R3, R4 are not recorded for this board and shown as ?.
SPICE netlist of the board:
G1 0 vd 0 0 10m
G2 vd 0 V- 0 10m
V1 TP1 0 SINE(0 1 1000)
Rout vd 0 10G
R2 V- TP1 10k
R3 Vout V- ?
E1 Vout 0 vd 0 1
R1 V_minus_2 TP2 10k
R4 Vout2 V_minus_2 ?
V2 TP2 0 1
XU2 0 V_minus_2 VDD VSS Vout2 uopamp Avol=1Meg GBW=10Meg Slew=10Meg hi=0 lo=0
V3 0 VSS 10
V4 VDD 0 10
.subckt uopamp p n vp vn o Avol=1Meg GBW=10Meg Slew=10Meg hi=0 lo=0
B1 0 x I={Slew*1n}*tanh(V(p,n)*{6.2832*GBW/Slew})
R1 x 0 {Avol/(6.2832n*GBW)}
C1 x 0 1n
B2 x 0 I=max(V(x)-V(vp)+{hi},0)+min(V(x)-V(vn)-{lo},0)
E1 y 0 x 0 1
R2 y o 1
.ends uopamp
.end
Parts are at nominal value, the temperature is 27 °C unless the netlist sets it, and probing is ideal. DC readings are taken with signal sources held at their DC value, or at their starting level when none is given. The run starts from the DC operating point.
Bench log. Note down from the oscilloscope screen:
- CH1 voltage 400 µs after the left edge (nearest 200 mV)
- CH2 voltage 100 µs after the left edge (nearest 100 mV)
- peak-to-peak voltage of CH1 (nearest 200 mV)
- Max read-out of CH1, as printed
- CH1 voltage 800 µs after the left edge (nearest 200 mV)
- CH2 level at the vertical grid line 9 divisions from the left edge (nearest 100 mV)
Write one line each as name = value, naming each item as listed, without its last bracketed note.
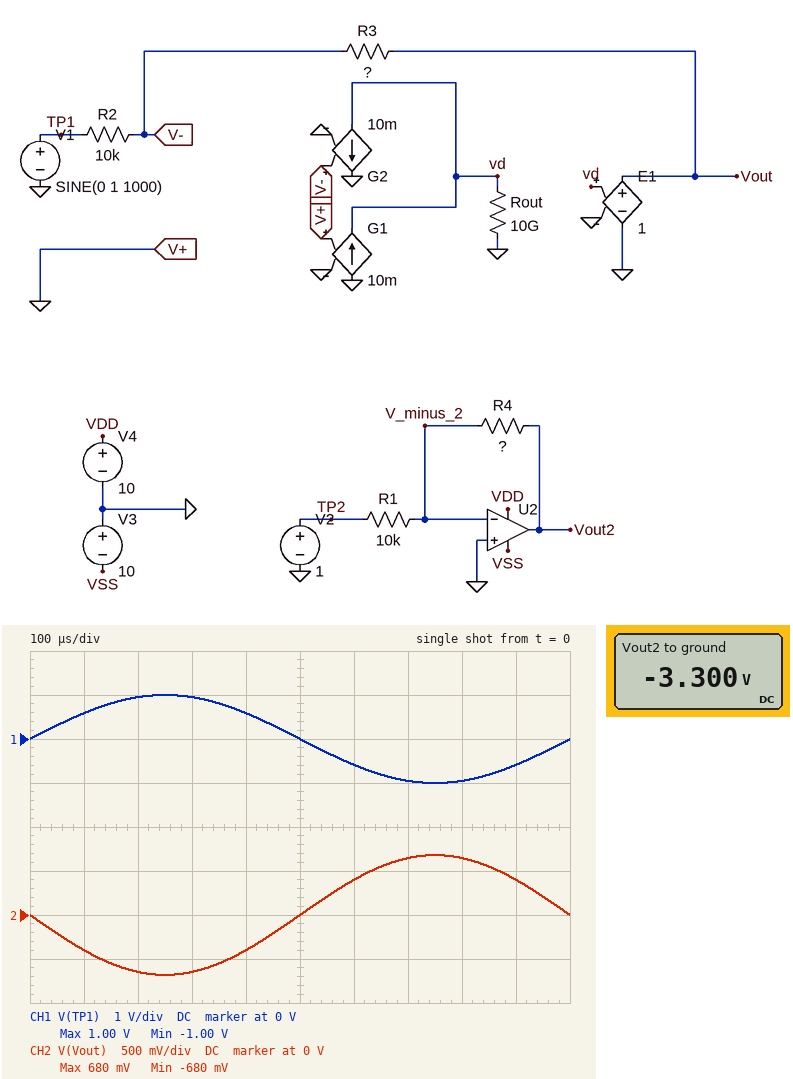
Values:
CH1 voltage 400 µs after the left edge = 600 mV
CH2 voltage 100 µs after the left edge = -400 mV
peak-to-peak voltage of CH1 = 2.0 V
Max read-out of CH1, as printed = 1.00 V
CH1 voltage 800 µs after the left edge = -1.0 V
CH2 level at the vertical grid line 9 divisions from the left edge = 400 mV
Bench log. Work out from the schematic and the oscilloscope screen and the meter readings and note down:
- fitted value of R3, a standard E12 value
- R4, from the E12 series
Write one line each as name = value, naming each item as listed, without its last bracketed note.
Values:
fitted value of R3, a standard E12 value = 6.8 kΩ
R4, from the E12 series = 33 kΩ
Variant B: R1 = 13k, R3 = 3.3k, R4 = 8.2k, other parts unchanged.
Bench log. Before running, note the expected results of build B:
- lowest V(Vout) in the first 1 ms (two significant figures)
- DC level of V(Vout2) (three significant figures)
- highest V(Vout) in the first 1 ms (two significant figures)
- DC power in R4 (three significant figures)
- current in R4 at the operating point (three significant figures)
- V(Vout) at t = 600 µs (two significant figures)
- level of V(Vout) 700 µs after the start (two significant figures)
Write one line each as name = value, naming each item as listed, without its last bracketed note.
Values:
lowest V(Vout) in the first 1 ms = -330 mV
DC level of V(Vout2) = -631 mV
highest V(Vout) in the first 1 ms = 330 mV
DC power in R4 = 48.5 µW
current in R4 at the operating point = 76.9 µA
V(Vout) at t = 600 µs = 190 mV
level of V(Vout) 700 µs after the start = 310 mV
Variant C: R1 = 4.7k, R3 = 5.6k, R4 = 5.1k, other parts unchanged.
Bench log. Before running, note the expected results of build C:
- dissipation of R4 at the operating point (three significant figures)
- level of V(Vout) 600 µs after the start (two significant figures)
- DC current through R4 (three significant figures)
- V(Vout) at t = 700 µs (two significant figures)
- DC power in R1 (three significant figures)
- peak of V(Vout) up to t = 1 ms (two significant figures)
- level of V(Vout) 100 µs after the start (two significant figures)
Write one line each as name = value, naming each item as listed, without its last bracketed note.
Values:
dissipation of R4 at the operating point = 231 µW
level of V(Vout) 600 µs after the start = 330 mV
DC current through R4 = 213 µA
V(Vout) at t = 700 µs = 530 mV
DC power in R1 = 213 µW
peak of V(Vout) up to t = 1 ms = 560 mV
level of V(Vout) 100 µs after the start = -330 mV
